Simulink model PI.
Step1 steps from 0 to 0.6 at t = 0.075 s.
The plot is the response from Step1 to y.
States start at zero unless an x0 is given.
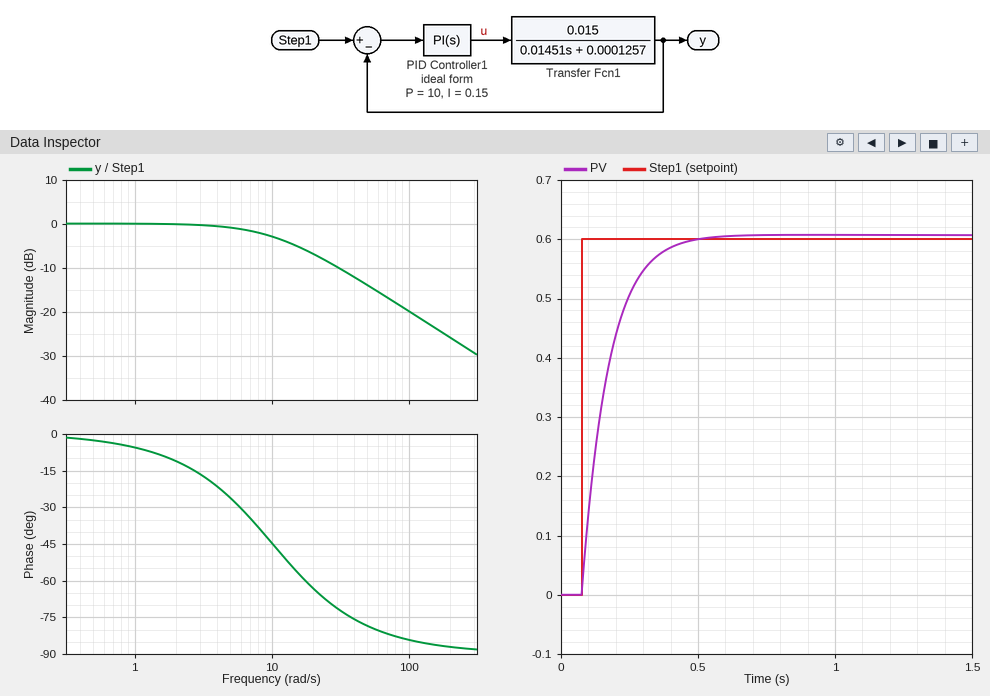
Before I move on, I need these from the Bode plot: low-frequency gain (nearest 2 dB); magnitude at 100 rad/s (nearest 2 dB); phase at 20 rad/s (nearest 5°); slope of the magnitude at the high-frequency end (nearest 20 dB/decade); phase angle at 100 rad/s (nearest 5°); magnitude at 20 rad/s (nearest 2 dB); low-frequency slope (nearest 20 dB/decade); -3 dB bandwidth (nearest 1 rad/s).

0 dB
-20 dB
-65°
-20 dB/decade
-85°
-6 dB
0 dB/decade
10 rad/s
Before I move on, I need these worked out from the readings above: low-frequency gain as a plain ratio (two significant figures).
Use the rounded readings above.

1.0
